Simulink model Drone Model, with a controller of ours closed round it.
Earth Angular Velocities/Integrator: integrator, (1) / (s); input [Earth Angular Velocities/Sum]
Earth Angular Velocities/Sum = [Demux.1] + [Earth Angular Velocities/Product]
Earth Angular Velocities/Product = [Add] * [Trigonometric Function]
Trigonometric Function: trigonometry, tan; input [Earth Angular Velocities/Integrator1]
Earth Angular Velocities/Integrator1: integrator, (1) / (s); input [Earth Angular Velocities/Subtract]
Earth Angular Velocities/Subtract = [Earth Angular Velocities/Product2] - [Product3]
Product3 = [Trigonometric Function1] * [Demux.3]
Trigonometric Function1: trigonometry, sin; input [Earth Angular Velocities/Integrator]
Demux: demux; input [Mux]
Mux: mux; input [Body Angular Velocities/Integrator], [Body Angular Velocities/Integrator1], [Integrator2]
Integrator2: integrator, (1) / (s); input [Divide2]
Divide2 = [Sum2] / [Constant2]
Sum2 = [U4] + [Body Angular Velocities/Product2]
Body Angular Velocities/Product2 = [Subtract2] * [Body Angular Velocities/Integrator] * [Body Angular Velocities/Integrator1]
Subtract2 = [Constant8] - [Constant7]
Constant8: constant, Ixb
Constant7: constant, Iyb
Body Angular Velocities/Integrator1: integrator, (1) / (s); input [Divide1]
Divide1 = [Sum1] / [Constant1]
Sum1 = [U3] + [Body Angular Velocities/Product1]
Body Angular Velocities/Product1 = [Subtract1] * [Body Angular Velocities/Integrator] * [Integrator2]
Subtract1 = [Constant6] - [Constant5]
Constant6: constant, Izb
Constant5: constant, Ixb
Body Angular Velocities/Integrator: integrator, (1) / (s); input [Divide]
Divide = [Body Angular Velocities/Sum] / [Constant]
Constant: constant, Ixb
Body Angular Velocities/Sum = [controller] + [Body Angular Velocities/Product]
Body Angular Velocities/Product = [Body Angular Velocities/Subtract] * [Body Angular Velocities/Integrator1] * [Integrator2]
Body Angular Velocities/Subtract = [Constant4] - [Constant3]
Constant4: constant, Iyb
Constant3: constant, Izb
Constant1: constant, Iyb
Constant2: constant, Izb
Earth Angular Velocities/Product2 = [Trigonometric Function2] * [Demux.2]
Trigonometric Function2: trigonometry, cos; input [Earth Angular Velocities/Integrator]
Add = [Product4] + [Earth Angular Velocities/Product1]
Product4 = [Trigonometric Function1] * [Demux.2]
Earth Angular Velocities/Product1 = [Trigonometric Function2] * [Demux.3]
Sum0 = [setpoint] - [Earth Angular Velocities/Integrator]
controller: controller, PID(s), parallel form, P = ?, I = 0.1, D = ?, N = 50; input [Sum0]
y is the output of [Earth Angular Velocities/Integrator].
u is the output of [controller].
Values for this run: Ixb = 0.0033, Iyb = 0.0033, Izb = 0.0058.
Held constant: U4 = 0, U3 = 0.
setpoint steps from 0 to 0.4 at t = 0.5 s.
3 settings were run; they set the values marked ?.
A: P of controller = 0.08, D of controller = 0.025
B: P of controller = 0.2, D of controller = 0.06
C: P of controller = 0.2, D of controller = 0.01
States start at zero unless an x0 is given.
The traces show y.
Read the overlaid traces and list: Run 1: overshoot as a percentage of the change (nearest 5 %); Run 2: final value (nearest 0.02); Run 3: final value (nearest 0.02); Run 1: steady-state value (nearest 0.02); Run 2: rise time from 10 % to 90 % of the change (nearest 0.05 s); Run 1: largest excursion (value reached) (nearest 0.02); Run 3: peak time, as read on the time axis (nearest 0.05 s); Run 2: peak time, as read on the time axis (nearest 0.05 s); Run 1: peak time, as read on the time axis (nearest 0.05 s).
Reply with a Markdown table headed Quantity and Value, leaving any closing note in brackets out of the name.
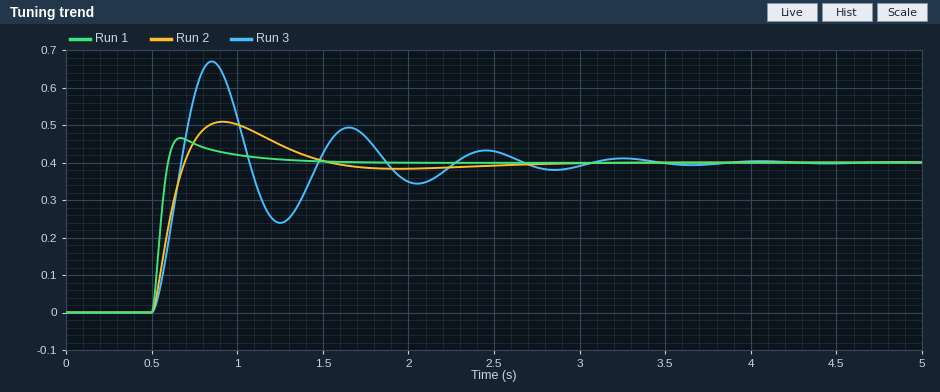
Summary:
| Quantity | Value |
|---|---|
| Run 1: overshoot as a percentage of the change | 15 % |
| Run 2: final value | 0.40 |
| Run 3: final value | 0.40 |
| Run 1: steady-state value | 0.40 |
| Run 2: rise time from 10 % to 90 % of the change | 0.15 s |
| Run 1: largest excursion (value reached) | 0.46 |
| Run 3: peak time, as read on the time axis | 0.85 s |
| Run 2: peak time, as read on the time axis | 0.90 s |
| Run 1: peak time, as read on the time axis | 0.65 s |
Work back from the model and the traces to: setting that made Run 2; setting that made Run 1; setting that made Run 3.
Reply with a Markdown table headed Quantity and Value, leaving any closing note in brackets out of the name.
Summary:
| Quantity | Value |
|---|---|
| setting that made Run 2 | A |
| setting that made Run 1 | B |
| setting that made Run 3 | C |
